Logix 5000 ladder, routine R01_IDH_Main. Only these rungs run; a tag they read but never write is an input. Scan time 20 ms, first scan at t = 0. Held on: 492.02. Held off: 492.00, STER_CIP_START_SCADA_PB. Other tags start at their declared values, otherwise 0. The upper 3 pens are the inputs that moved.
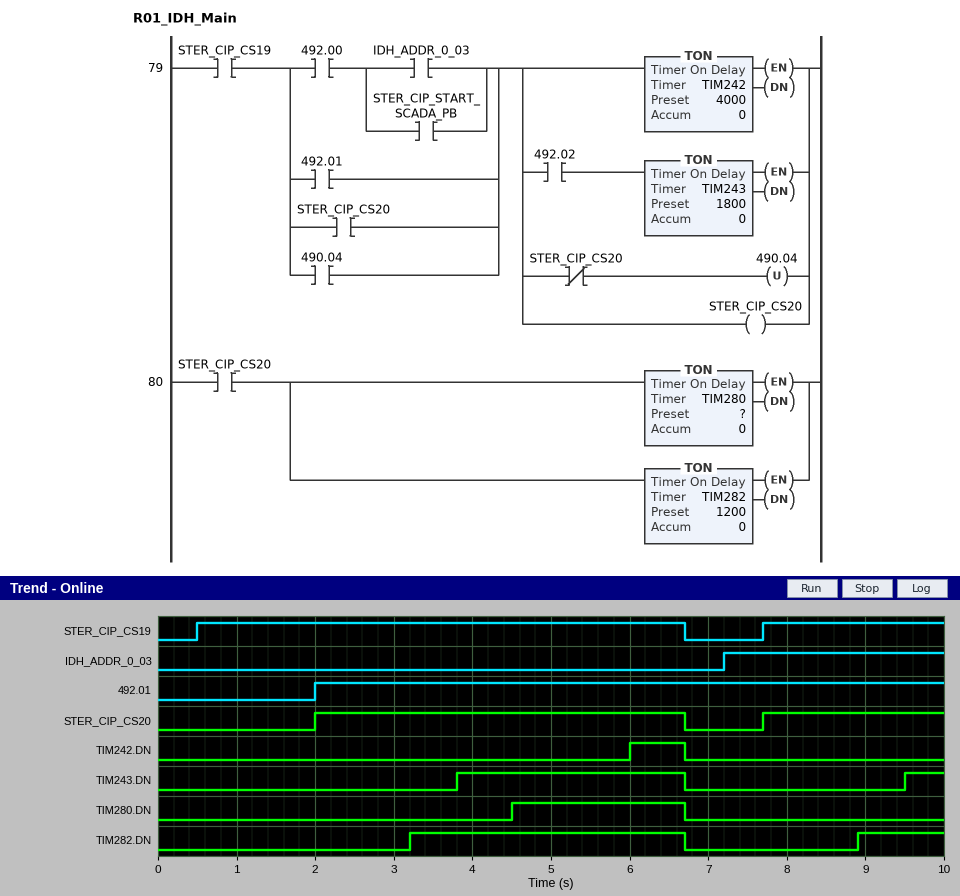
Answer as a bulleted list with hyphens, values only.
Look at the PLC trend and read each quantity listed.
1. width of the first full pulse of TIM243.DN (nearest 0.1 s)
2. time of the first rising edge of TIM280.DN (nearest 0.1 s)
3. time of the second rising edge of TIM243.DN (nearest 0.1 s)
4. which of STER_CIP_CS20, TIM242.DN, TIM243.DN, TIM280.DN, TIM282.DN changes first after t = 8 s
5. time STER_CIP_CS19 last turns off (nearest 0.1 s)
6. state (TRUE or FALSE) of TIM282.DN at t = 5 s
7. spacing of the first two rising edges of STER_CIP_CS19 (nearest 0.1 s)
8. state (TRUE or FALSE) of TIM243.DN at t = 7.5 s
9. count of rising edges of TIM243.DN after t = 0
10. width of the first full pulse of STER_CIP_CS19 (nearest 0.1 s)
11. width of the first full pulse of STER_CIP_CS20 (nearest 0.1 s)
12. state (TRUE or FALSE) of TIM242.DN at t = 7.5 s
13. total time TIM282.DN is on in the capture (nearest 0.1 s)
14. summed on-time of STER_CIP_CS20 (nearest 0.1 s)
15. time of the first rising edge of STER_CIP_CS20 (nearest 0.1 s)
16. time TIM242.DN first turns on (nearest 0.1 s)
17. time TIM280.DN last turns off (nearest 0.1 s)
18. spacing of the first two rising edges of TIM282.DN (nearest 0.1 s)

- 2.9 s
- 4.5 s
- 9.5 s
- TIM282.DN
- 6.7 s
- TRUE
- 7.2 s
- FALSE
- 2
- 6.2 s
- 4.7 s
- FALSE
- 4.6 s
- 7.0 s
- 2.0 s
- 6.0 s
- 6.7 s
- 5.7 s
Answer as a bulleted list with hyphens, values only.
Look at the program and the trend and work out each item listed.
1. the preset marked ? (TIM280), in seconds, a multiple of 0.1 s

- 2.5 s
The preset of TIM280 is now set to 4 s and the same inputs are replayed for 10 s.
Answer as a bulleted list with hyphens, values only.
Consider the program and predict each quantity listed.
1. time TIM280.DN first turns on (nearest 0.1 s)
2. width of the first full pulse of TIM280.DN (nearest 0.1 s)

- 6.0 s
- 0.7 s
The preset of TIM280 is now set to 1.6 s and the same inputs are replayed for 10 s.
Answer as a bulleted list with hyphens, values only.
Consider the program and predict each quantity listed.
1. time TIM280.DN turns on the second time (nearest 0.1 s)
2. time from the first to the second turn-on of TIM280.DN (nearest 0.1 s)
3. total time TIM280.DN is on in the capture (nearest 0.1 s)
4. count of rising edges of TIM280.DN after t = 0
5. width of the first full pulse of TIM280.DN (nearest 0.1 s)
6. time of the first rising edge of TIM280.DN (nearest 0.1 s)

- 9.3 s
- 5.7 s
- 3.8 s
- 2
- 3.1 s
- 3.6 s
